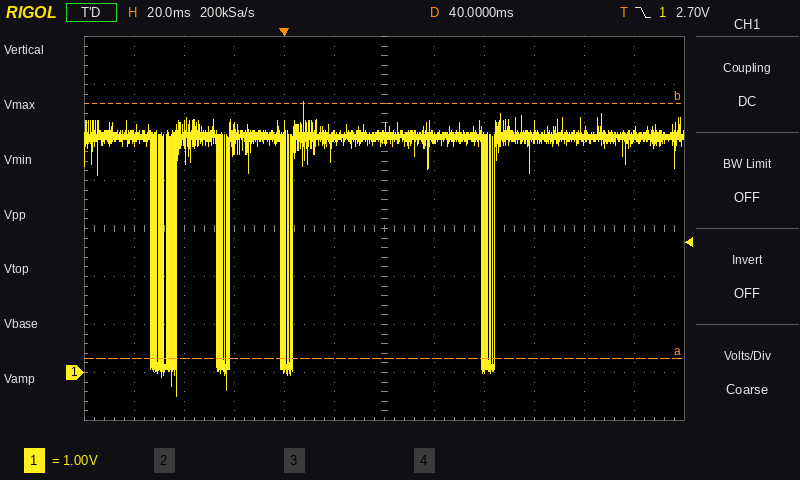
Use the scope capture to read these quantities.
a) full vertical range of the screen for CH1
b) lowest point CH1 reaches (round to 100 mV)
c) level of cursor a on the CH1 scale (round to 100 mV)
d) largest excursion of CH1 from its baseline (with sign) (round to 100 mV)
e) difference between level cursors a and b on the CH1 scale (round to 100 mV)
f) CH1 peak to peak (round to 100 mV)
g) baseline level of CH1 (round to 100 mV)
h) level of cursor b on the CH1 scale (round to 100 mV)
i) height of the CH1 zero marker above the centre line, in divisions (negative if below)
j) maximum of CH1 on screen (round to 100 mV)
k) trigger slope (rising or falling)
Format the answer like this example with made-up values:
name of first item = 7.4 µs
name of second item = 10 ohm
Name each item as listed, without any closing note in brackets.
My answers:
full vertical range of the screen for CH1 = 8 V
lowest point CH1 reaches = -500 mV
level of cursor a on the CH1 scale = 300 mV
largest excursion of CH1 from its baseline (with sign) = -5.4 V
difference between level cursors a and b on the CH1 scale = 5.3 V
CH1 peak to peak = 6.1 V
baseline level of CH1 = 4.9 V
level of cursor b on the CH1 scale = 5.6 V
height of the CH1 zero marker above the centre line, in divisions = -3.0 div
maximum of CH1 on screen = 5.6 V
trigger slope = falling
